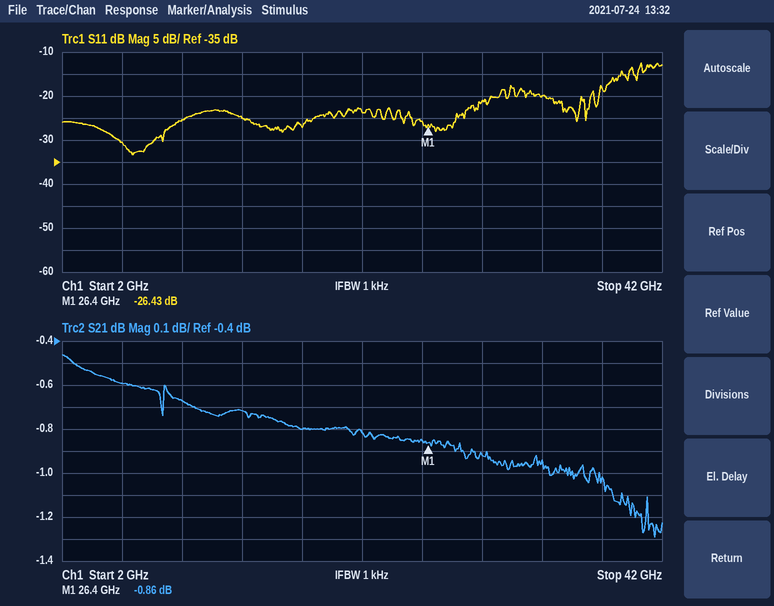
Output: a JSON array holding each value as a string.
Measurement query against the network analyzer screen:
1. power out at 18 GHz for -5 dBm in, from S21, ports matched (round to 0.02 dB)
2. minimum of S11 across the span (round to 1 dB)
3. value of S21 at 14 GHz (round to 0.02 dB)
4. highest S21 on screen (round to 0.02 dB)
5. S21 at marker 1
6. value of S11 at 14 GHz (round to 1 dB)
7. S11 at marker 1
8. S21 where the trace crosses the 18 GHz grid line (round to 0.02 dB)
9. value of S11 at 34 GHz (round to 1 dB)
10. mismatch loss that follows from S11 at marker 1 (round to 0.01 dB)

["-5.80 dBm", "-33 dB", "-0.72 dB", "-0.46 dB", "-0.86 dB", "-25 dB", "-26.43 dB", "-0.80 dB", "-20 dB", "0.01 dB"]
